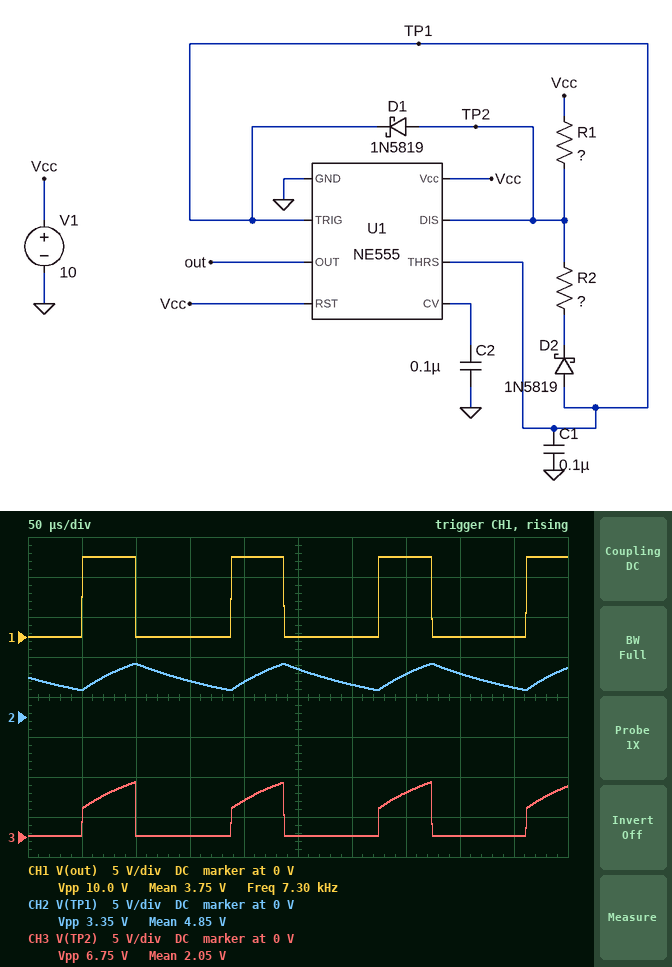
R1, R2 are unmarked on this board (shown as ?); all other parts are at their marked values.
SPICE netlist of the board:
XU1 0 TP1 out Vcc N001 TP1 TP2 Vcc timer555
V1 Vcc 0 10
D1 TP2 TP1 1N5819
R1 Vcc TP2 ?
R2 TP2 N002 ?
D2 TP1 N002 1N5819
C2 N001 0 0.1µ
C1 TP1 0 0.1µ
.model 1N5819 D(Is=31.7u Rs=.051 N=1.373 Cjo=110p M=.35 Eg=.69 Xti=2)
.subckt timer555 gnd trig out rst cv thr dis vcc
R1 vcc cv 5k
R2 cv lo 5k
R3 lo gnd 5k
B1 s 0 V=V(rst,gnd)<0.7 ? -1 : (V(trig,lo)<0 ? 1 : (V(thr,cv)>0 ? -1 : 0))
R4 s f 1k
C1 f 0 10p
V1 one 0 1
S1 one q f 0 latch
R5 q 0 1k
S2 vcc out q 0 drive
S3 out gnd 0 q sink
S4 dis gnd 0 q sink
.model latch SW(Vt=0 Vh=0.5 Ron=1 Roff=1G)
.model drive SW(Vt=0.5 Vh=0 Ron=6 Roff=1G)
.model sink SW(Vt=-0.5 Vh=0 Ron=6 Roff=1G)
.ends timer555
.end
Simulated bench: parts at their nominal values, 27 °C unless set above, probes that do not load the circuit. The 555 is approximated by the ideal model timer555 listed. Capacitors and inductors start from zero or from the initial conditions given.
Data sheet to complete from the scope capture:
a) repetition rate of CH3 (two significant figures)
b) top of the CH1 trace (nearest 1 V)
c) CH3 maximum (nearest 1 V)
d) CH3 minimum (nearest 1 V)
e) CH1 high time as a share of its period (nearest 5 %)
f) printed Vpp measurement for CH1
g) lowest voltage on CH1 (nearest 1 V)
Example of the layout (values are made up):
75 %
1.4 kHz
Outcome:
7.3 kHz
10 V
7 V
0 V
35 %
10.0 V
0 V
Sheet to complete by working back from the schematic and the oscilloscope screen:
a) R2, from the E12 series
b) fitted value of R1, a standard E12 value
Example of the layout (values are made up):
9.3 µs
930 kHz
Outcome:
1.2 kΩ
680 Ω
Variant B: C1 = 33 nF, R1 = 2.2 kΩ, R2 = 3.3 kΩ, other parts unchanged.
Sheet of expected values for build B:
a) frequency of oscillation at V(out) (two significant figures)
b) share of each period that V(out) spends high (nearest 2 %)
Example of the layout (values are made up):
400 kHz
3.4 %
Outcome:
7.8 kHz
40 %
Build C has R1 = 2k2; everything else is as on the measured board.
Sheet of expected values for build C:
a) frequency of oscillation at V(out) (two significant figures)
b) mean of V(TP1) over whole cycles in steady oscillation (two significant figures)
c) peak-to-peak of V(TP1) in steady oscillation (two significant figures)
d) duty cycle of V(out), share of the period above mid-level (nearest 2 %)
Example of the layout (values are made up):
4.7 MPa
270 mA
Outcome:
4.1 kHz
5.1 V
3.3 V
64 %
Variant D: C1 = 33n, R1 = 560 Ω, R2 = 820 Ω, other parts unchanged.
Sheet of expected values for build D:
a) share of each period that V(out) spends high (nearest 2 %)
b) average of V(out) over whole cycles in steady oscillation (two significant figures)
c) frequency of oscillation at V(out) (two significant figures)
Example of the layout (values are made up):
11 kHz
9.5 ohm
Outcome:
40 %
4.0 V
30 kHz
